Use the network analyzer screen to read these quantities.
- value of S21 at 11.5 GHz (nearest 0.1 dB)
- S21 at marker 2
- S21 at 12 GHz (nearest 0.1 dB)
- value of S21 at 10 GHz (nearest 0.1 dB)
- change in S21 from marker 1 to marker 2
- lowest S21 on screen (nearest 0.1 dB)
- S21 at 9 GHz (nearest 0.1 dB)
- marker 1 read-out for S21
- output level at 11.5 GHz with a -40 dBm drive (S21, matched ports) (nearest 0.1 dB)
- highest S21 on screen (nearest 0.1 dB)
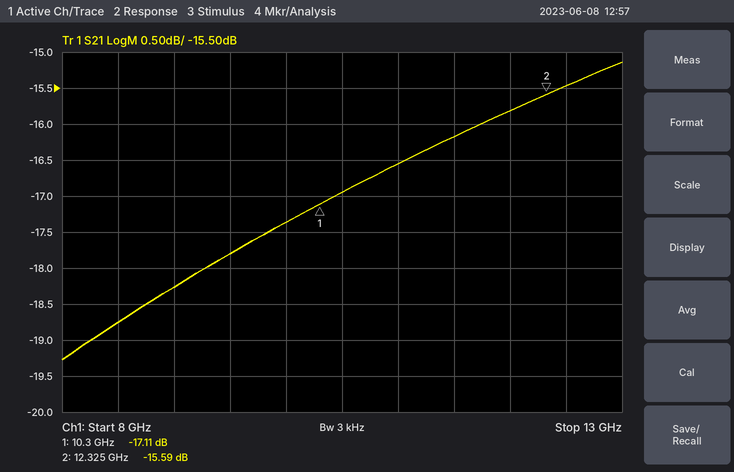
-16.2 dB
-15.59 dB
-15.8 dB
-17.4 dB
1.52 dB
-19.3 dB
-18.3 dB
-17.11 dB
-56.2 dBm
-15.1 dB
